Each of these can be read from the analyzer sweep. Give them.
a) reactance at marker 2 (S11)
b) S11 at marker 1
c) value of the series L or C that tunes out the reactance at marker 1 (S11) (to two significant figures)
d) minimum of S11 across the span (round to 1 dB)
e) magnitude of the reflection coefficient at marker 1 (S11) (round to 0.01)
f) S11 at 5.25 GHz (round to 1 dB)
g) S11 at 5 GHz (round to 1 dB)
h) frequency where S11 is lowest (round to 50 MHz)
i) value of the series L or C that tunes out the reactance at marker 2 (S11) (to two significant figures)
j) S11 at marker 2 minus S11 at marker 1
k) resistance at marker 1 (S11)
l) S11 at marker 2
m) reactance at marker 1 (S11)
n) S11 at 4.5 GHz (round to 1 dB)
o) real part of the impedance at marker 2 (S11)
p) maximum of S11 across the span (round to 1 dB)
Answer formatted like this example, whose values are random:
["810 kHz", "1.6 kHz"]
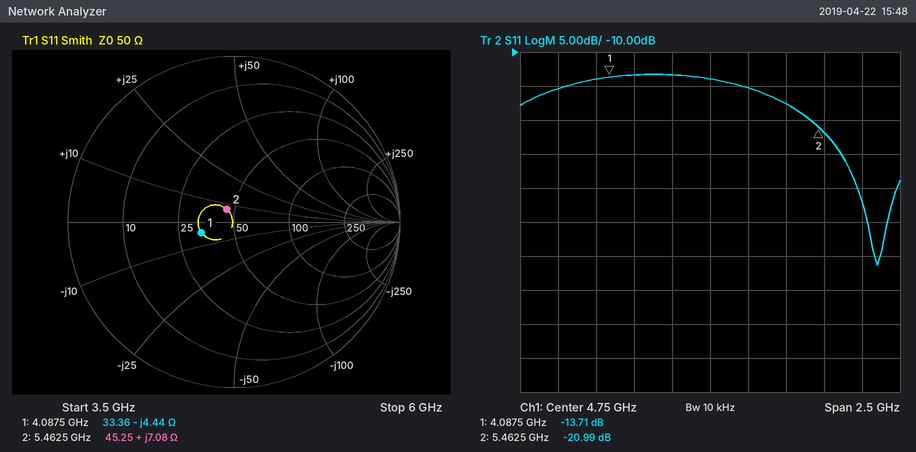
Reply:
["+7.08 Ω", "-13.71 dB", "170 pH", "-41 dB", "0.21", "-18 dB", "-15 dB", "5.85 GHz", "4.1 pF", "-7.28 dB", "33.36 Ω", "-20.99 dB", "-4.44 Ω", "-13 dB", "45.25 Ω", "-13 dB"]
